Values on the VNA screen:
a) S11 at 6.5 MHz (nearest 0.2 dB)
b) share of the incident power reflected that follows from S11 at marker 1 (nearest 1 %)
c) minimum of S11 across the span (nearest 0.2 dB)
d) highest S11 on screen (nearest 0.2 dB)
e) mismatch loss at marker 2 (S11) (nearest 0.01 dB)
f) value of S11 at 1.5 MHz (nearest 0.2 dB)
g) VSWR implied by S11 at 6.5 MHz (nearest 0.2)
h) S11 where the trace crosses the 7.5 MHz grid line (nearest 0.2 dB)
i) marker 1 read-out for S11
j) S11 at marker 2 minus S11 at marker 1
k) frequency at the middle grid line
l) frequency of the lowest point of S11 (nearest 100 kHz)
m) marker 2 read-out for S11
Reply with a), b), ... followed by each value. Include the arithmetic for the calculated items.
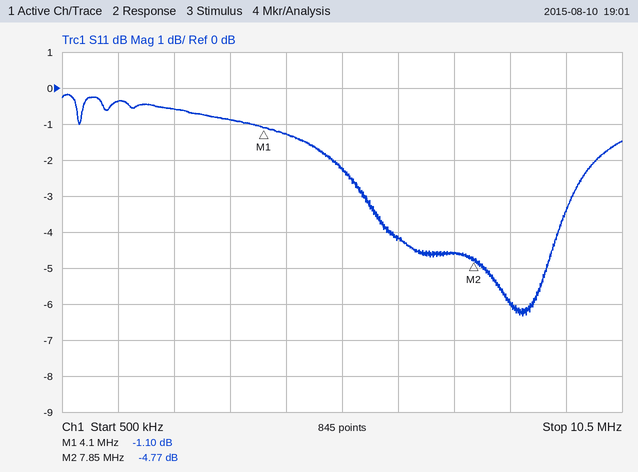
a) -4.2 dB
b) 10^(-1.1/10) ≈ 78 %
c) -6.4 dB
d) -0.2 dB
e) −10 log10(1 − 10^(-4.77/10)) ≈ 1.76 dB
f) -0.4 dB
g) |Γ| = 10^(-4.2/20) = 0.6166; VSWR = (1 + 0.6166)/(1 − 0.6166) ≈ 4.2
h) -4.6 dB
i) -1.10 dB
j) -4.77 − (-1.1) = -3.67 dB
k) 5.5 MHz
l) 8.7 MHz
m) -4.77 dB
